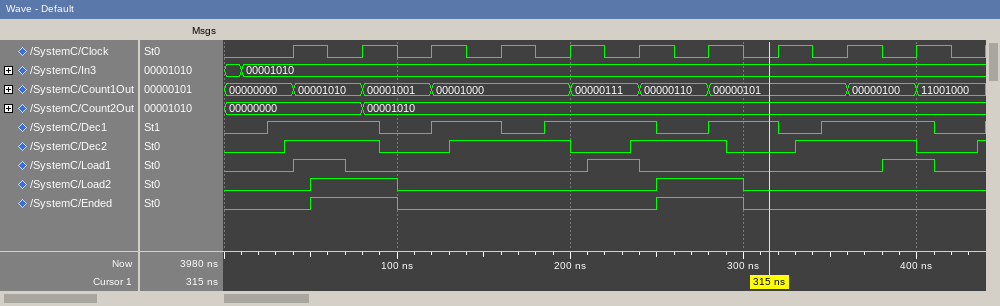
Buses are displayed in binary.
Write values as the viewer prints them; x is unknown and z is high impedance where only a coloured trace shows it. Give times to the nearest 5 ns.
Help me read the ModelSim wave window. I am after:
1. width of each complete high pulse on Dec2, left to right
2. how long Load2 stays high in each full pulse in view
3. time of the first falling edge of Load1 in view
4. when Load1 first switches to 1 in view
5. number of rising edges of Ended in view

55 ns, 70 ns, 55 ns, 70 ns
50 ns, 50 ns
70 ns
40 ns
2
